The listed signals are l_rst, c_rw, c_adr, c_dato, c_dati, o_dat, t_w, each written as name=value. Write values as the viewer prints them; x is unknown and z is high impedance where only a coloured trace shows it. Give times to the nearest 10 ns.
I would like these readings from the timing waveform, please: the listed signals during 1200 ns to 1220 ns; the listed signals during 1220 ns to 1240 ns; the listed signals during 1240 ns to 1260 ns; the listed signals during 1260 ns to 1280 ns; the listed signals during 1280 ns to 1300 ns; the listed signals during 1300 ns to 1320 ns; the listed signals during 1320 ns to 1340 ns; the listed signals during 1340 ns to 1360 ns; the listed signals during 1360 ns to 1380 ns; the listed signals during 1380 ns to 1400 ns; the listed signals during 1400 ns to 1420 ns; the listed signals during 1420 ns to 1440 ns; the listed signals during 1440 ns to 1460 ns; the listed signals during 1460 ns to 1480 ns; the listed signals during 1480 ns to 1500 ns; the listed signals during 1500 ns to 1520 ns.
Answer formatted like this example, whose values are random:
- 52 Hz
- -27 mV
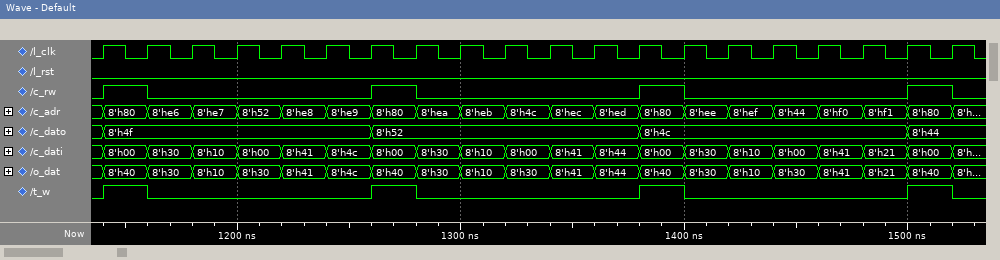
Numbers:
- l_rst=0, c_rw=0, c_adr=8'h52, c_dato=8'h4f, c_dati=8'h00, o_dat=8'h30, t_w=0
- l_rst=0, c_rw=0, c_adr=8'he8, c_dato=8'h4f, c_dati=8'h41, o_dat=8'h41, t_w=0
- l_rst=0, c_rw=0, c_adr=8'he9, c_dato=8'h4f, c_dati=8'h4c, o_dat=8'h4c, t_w=0
- l_rst=0, c_rw=1, c_adr=8'h80, c_dato=8'h52, c_dati=8'h00, o_dat=8'h40, t_w=1
- l_rst=0, c_rw=0, c_adr=8'hea, c_dato=8'h52, c_dati=8'h30, o_dat=8'h30, t_w=0
- l_rst=0, c_rw=0, c_adr=8'heb, c_dato=8'h52, c_dati=8'h10, o_dat=8'h10, t_w=0
- l_rst=0, c_rw=0, c_adr=8'h4c, c_dato=8'h52, c_dati=8'h00, o_dat=8'h30, t_w=0
- l_rst=0, c_rw=0, c_adr=8'hec, c_dato=8'h52, c_dati=8'h41, o_dat=8'h41, t_w=0
- l_rst=0, c_rw=0, c_adr=8'hed, c_dato=8'h52, c_dati=8'h44, o_dat=8'h44, t_w=0
- l_rst=0, c_rw=1, c_adr=8'h80, c_dato=8'h4c, c_dati=8'h00, o_dat=8'h40, t_w=1
- l_rst=0, c_rw=0, c_adr=8'hee, c_dato=8'h4c, c_dati=8'h30, o_dat=8'h30, t_w=0
- l_rst=0, c_rw=0, c_adr=8'hef, c_dato=8'h4c, c_dati=8'h10, o_dat=8'h10, t_w=0
- l_rst=0, c_rw=0, c_adr=8'h44, c_dato=8'h4c, c_dati=8'h00, o_dat=8'h30, t_w=0
- l_rst=0, c_rw=0, c_adr=8'hf0, c_dato=8'h4c, c_dati=8'h41, o_dat=8'h41, t_w=0
- l_rst=0, c_rw=0, c_adr=8'hf1, c_dato=8'h4c, c_dati=8'h21, o_dat=8'h21, t_w=0
- l_rst=0, c_rw=1, c_adr=8'h80, c_dato=8'h44, c_dati=8'h00, o_dat=8'h40, t_w=1
